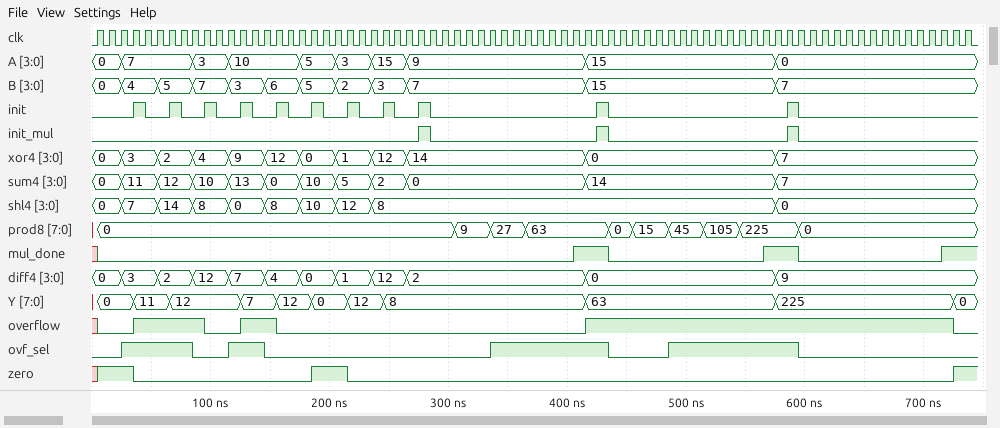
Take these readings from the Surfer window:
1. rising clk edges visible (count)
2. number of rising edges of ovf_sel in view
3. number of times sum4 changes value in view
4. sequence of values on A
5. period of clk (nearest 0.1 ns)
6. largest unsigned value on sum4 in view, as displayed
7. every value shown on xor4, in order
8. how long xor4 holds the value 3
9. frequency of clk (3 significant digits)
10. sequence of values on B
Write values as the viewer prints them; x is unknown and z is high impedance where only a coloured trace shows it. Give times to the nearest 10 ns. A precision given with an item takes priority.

74
4
11
0, 7, 3, 10, 5, 3, 15, 9, 15, 0
10 ns
14
0, 3, 2, 4, 9, 12, 0, 1, 12, 14, 0, 7
30 ns
100 MHz
0, 4, 5, 7, 3, 6, 5, 2, 3, 7, 15, 7
